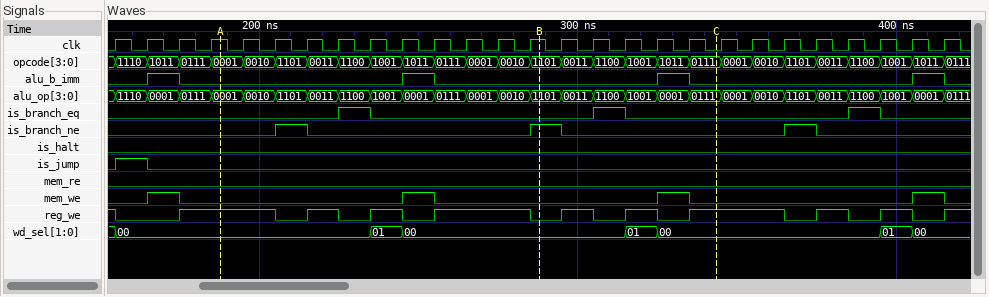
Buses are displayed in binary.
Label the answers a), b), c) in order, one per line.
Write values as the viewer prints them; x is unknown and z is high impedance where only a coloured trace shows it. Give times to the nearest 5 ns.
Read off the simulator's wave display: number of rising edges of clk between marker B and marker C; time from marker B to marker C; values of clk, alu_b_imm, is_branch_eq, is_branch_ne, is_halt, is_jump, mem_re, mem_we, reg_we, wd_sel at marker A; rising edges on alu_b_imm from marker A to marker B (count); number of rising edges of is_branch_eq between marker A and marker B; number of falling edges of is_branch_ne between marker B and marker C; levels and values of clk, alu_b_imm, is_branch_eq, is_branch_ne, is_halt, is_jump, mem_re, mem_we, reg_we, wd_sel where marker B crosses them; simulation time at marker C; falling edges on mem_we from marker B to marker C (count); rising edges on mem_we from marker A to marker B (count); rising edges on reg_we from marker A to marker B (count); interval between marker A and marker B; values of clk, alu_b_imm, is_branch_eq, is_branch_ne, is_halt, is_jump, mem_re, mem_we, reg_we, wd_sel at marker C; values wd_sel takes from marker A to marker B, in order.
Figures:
a) 5
b) 55 ns
c) clk=1, alu_b_imm=0, is_branch_eq=0, is_branch_ne=0, is_halt=0, is_jump=0, mem_re=0, mem_we=0, reg_we=1, wd_sel=00
d) 1
e) 1
f) 1
g) clk=1, alu_b_imm=0, is_branch_eq=0, is_branch_ne=1, is_halt=0, is_jump=0, mem_re=0, mem_we=0, reg_we=0, wd_sel=00
h) 345 ns
i) 1
j) 1
k) 3
l) 100 ns
m) clk=0, alu_b_imm=0, is_branch_eq=0, is_branch_ne=0, is_halt=0, is_jump=0, mem_re=0, mem_we=0, reg_we=1, wd_sel=00
n) 00, 01, 00
